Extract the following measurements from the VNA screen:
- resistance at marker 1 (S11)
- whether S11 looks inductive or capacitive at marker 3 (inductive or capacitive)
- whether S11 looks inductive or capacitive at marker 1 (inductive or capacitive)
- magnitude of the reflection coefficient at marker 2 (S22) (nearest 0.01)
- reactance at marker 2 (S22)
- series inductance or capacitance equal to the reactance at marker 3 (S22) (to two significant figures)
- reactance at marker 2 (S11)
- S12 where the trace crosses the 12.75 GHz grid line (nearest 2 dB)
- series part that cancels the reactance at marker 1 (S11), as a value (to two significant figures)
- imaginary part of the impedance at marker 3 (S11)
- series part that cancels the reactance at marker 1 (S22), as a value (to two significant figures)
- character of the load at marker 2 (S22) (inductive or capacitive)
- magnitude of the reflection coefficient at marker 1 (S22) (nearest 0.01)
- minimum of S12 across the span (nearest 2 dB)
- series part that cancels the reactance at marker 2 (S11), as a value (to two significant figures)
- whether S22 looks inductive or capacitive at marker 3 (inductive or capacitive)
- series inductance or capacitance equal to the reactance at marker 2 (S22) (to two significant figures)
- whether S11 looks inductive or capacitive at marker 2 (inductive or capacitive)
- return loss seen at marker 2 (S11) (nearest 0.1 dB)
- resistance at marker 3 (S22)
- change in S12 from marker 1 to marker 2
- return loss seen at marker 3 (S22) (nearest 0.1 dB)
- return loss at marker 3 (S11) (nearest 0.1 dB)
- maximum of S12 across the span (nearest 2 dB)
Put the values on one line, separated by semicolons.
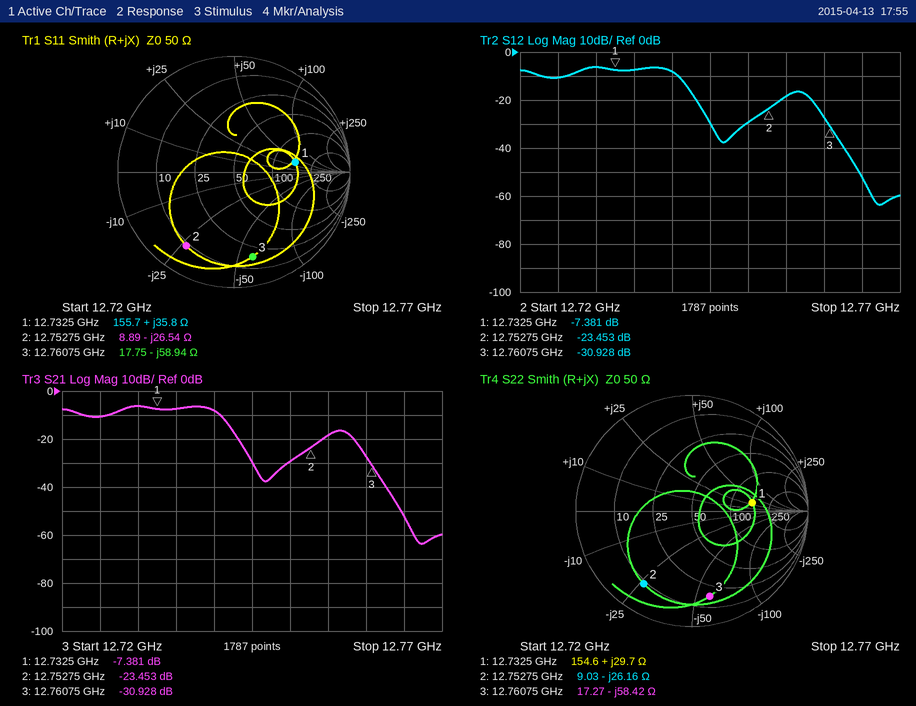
155.7 Ω; capacitive; inductive; 0.75; -26.16 Ω; 210 fF; -26.54 Ω; -30 dB; 350 fF; -58.94 Ω; 420 fF; capacitive; 0.53; -64 dB; 330 pH; capacitive; 480 fF; capacitive; 2.4 dB; 17.27 Ω; -16.072 dB; 2.5 dB; 2.5 dB; -6 dB
